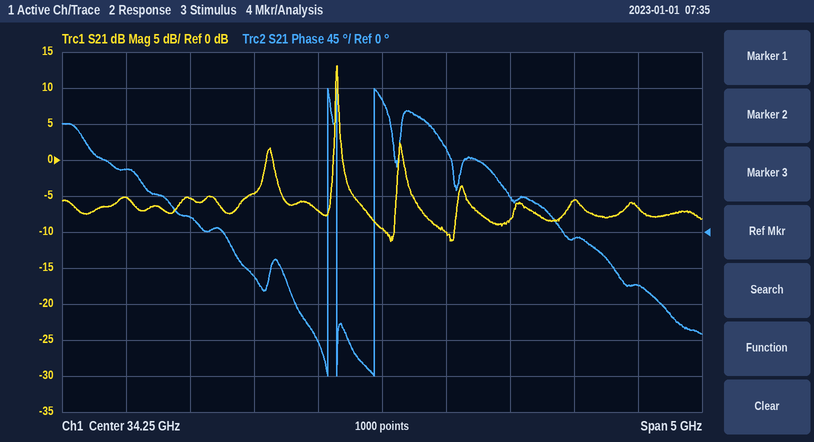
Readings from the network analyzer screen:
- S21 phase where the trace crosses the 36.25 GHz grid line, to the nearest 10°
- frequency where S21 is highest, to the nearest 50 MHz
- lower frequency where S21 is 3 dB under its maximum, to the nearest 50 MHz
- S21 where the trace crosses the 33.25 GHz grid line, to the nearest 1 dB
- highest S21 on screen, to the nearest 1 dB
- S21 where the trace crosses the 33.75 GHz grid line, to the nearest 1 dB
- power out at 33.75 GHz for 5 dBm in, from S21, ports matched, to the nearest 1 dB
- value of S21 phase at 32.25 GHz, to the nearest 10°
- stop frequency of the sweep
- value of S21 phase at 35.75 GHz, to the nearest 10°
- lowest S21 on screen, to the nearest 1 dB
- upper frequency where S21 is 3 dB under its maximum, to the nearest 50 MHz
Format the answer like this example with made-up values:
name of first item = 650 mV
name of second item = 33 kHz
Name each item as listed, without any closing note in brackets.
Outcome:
S21 phase where the trace crosses the 36.25 GHz grid line, to the nearest 10° = -70°
frequency where S21 is highest, to the nearest 50 MHz = 33.90 GHz
lower frequency where S21 is 3 dB under its maximum, to the nearest 50 MHz = 33.90 GHz
S21 where the trace crosses the 33.25 GHz grid line, to the nearest 1 dB = -5 dB
highest S21 on screen, to the nearest 1 dB = 13 dB
S21 where the trace crosses the 33.75 GHz grid line, to the nearest 1 dB = -7 dB
power out at 33.75 GHz for 5 dBm in, from S21, ports matched, to the nearest 1 dB = -2 dBm
value of S21 phase at 32.25 GHz, to the nearest 10° = 80°
stop frequency of the sweep = 36.75 GHz
value of S21 phase at 35.75 GHz, to the nearest 10° = -10°
lowest S21 on screen, to the nearest 1 dB = -11 dB
upper frequency where S21 is 3 dB under its maximum, to the nearest 50 MHz = 33.90 GHz
